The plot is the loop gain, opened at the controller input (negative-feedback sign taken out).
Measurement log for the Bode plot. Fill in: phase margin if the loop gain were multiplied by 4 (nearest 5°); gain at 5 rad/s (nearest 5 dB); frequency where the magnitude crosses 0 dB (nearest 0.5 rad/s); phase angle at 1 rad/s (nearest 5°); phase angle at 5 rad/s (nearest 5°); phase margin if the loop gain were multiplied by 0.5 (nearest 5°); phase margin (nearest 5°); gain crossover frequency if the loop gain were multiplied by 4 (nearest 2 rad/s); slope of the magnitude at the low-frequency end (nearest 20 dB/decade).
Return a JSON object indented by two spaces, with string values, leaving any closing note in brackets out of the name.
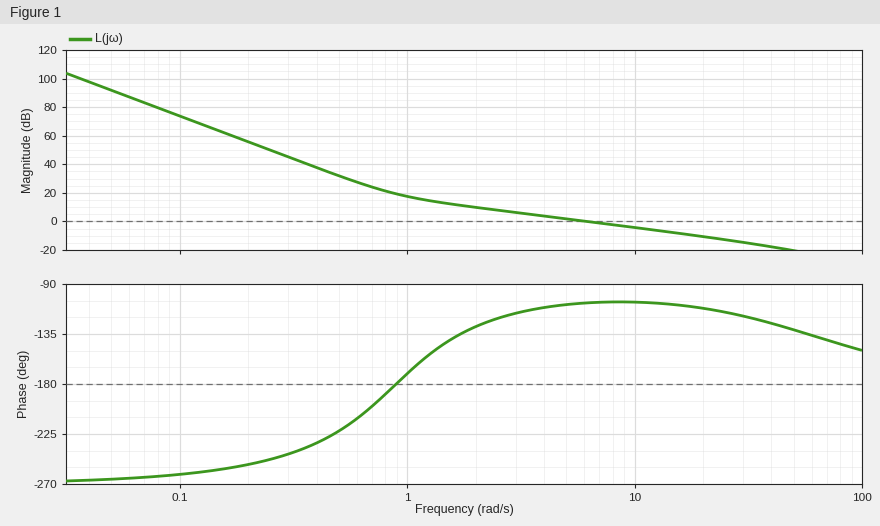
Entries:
{
  "phase margin if the loop gain were multiplied by 4": "65°",
  "gain at 5 rad/s": "0 dB",
  "frequency where the magnitude crosses 0 dB": "6.0 rad/s",
  "phase angle at 1 rad/s": "-170°",
  "phase angle at 5 rad/s": "-110°",
  "phase margin if the loop gain were multiplied by 0.5": "65°",
  "phase margin": "75°",
  "gain crossover frequency if the loop gain were multiplied by 4": "24 rad/s",
  "slope of the magnitude at the low-frequency end": "-60 dB/decade"
}
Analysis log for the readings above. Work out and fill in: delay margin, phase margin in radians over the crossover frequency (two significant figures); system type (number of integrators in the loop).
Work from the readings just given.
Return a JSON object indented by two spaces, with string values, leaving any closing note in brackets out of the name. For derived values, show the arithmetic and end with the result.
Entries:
{
  "delay margin, phase margin in radians over the crossover frequency": "75 × π / 180 / 6 = 0.22 s",
  "system type": "3"
}
